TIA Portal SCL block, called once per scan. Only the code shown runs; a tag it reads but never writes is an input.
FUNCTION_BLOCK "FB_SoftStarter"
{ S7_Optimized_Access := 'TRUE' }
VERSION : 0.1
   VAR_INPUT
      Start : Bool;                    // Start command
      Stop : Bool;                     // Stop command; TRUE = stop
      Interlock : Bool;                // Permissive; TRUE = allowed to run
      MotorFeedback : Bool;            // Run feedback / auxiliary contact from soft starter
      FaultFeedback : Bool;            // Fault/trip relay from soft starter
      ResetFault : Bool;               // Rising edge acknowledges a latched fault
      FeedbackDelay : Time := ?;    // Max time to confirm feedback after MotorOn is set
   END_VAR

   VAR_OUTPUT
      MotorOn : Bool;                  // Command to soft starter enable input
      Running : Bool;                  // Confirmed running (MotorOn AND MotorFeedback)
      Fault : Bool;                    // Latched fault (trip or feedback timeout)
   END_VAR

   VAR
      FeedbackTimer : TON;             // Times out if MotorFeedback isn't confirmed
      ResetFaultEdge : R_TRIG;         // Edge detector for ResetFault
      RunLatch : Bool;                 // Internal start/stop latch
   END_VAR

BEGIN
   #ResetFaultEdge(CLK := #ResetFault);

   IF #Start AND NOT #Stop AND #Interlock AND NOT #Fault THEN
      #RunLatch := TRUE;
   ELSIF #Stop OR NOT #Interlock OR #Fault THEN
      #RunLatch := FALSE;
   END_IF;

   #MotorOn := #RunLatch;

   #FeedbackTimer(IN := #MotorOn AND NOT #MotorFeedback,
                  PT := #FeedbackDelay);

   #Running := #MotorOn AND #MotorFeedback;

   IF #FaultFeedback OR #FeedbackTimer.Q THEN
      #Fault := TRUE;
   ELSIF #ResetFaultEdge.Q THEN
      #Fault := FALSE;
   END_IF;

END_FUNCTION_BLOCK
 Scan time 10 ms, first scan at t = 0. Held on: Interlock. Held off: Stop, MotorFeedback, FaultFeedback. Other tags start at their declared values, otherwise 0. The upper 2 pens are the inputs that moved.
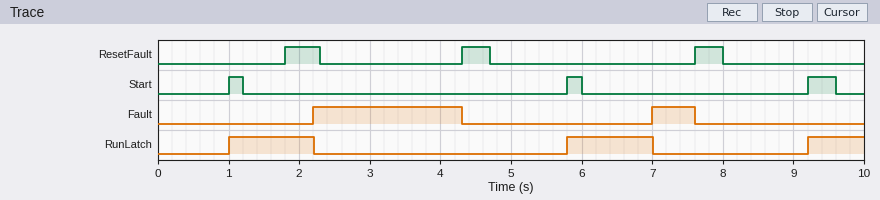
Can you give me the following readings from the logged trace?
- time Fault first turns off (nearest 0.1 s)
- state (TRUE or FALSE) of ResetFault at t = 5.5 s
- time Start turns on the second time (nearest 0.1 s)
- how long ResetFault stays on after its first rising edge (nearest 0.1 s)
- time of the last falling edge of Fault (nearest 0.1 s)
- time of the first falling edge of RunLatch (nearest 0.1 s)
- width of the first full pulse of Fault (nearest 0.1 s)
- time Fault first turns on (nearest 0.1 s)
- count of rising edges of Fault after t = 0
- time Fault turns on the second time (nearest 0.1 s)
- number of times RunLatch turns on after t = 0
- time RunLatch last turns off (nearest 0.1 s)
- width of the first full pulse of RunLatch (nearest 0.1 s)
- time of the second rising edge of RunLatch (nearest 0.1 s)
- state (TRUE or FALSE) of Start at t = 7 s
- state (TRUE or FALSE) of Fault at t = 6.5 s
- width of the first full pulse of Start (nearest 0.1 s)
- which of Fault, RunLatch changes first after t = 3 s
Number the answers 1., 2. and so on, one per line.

1. 4.3 s
2. FALSE
3. 5.8 s
4. 0.5 s
5. 7.6 s
6. 2.2 s
7. 2.1 s
8. 2.2 s
9. 2
10. 7.0 s
11. 3
12. 7.0 s
13. 1.2 s
14. 5.8 s
15. FALSE
16. FALSE
17. 0.2 s
18. Fault
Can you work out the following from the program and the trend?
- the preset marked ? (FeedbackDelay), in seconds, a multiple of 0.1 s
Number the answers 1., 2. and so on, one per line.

1. 1.2 s
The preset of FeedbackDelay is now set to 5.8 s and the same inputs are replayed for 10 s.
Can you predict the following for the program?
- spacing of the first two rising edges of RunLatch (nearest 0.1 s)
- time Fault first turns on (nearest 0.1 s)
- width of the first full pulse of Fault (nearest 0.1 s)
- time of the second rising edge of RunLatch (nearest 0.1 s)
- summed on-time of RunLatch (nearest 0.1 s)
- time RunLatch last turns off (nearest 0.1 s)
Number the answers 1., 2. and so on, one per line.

1. 8.2 s
2. 6.8 s
3. 0.8 s
4. 9.2 s
5. 6.6 s
6. 6.8 s
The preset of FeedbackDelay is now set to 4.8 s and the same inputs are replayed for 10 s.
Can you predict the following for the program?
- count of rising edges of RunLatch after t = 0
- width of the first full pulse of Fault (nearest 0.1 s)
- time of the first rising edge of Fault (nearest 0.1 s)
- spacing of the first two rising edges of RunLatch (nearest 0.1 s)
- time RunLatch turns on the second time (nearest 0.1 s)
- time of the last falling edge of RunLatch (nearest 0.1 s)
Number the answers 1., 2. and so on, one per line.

1. 2
2. 1.8 s
3. 5.8 s
4. 8.2 s
5. 9.2 s
6. 5.8 s
